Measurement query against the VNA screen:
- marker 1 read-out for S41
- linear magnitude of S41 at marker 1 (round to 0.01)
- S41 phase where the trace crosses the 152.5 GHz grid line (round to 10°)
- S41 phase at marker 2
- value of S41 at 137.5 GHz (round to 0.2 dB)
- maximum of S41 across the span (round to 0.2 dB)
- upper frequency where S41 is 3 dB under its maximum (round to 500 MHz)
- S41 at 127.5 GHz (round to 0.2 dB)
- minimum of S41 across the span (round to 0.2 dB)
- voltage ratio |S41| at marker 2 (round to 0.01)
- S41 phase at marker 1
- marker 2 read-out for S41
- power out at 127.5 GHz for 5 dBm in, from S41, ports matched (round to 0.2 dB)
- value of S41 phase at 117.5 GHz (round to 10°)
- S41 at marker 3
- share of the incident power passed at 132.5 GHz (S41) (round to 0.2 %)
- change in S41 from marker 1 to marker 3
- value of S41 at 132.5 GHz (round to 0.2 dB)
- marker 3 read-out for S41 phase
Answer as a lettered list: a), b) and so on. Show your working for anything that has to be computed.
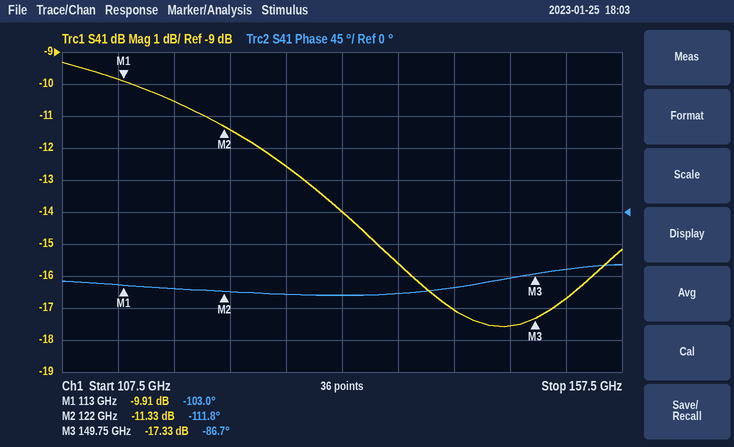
a) -9.91 dB
b) 10^(-9.91/20) ≈ 0.32
c) -80°
d) -111.8°
e) -15.6 dB
f) -9.4 dB
g) 126.5 GHz
h) -12.6 dB
i) -17.6 dB
j) 10^(-11.33/20) ≈ 0.27
k) -103.0°
l) -11.33 dB
m) 5 dBm + (-12.6 dB) = -7.6 dBm
n) -110°
o) -17.33 dB
p) 10^(-14/10) ≈ 4.0 %
q) -17.33 − (-9.91) = -7.42 dB
r) -14.0 dB
s) -86.7°
